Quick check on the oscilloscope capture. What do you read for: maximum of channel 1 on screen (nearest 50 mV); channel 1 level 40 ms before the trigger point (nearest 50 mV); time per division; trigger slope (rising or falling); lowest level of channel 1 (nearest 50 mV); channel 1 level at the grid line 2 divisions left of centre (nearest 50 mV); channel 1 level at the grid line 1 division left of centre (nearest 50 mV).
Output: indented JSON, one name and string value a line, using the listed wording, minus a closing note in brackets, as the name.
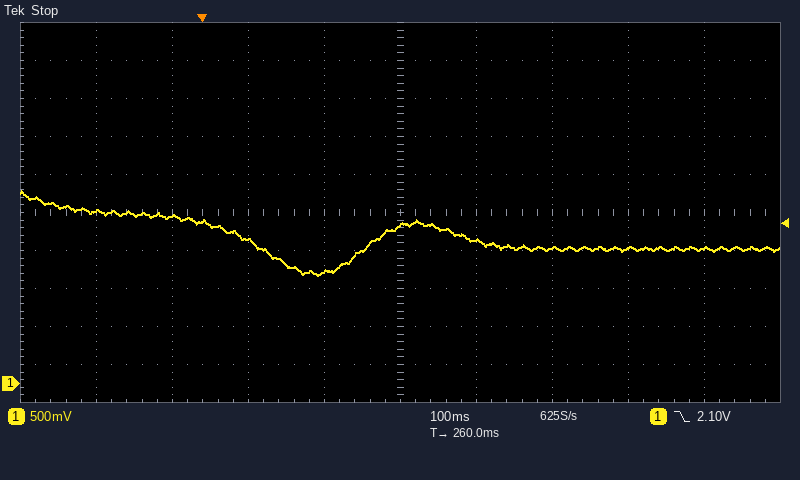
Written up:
{
  "maximum of channel 1 on screen": "2.55 V",
  "channel 1 level 40 ms before the trigger point": "2.20 V",
  "time per division": "100 ms",
  "trigger slope": "falling",
  "lowest level of channel 1": "1.40 V",
  "channel 1 level at the grid line 2 divisions left of centre": "1.90 V",
  "channel 1 level at the grid line 1 division left of centre": "1.45 V"
}
